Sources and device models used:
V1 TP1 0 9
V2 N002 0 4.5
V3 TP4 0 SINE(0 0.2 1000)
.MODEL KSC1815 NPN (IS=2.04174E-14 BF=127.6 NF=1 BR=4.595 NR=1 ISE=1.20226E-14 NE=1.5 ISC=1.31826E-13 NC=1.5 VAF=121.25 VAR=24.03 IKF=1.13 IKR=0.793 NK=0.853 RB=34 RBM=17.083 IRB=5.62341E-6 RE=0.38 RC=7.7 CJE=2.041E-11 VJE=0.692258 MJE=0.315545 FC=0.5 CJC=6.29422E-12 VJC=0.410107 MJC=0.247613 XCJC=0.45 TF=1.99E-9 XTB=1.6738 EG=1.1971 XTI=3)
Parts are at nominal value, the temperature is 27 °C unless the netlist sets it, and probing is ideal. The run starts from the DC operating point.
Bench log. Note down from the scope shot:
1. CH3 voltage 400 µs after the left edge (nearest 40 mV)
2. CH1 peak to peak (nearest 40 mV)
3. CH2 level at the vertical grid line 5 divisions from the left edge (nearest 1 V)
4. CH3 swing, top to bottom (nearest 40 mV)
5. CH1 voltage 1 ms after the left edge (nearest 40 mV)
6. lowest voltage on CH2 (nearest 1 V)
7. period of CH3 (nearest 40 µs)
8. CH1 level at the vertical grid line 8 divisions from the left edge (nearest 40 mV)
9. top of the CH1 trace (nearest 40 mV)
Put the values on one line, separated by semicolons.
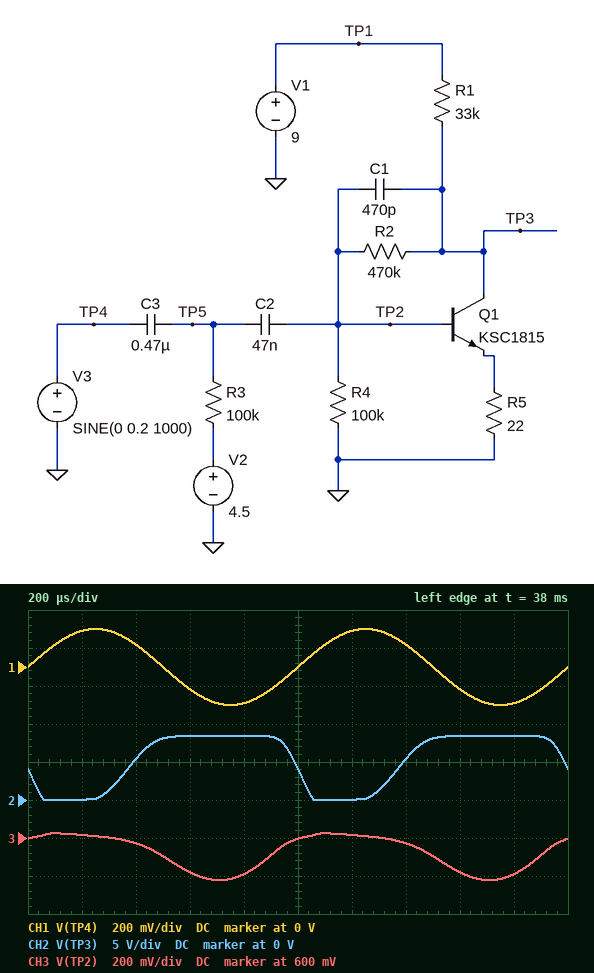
560 mV; 400 mV; 4 V; 240 mV; 0 V; 0 V; 1.00 ms; -120 mV; 200 mV
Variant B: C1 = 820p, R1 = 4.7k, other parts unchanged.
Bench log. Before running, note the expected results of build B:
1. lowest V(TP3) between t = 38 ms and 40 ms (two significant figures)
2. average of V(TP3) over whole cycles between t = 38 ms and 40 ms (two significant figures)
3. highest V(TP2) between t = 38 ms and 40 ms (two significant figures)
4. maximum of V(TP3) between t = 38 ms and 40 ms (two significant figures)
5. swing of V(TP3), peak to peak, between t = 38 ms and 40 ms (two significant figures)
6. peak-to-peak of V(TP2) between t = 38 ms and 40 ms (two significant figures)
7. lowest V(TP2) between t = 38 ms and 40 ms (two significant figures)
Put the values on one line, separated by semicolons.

910 mV; 5.9 V; 690 mV; 8.9 V; 8.0 V; 220 mV; 470 mV
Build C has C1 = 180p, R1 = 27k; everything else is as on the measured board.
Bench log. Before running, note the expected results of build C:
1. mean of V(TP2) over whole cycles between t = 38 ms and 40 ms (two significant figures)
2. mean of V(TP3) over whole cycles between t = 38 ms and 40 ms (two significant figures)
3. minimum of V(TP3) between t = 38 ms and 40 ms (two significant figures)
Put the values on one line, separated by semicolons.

510 mV; 5.6 V; 42 mV
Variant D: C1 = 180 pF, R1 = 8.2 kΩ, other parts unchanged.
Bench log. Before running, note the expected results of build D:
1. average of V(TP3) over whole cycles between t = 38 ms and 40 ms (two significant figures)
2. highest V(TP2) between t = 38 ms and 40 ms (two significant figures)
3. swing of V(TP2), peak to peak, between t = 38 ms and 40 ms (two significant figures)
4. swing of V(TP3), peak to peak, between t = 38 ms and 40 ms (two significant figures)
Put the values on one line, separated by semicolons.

5.9 V; 670 mV; 290 mV; 8.8 V
